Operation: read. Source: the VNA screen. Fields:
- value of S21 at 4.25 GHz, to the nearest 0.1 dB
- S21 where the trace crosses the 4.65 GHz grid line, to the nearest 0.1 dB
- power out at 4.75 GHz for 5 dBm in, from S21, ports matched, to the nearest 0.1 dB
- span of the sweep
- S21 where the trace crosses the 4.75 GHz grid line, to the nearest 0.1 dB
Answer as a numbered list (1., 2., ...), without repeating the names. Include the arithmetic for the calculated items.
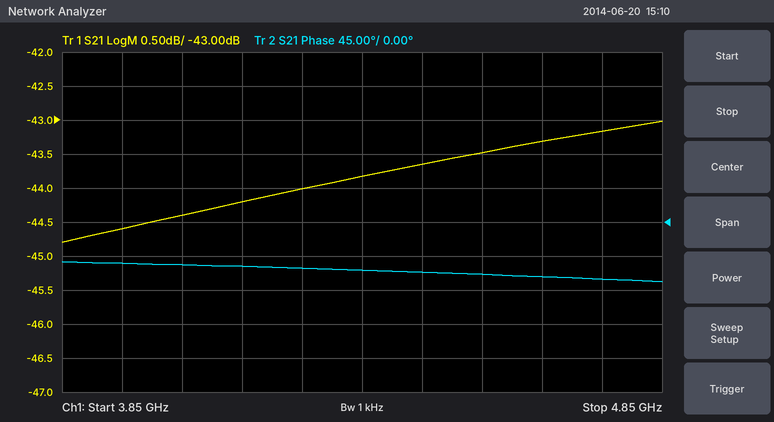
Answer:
1. -44.0 dB
2. -43.3 dB
3. 5 dBm + (-43.2 dB) = -38.2 dBm
4. 1 GHz
5. -43.2 dB
